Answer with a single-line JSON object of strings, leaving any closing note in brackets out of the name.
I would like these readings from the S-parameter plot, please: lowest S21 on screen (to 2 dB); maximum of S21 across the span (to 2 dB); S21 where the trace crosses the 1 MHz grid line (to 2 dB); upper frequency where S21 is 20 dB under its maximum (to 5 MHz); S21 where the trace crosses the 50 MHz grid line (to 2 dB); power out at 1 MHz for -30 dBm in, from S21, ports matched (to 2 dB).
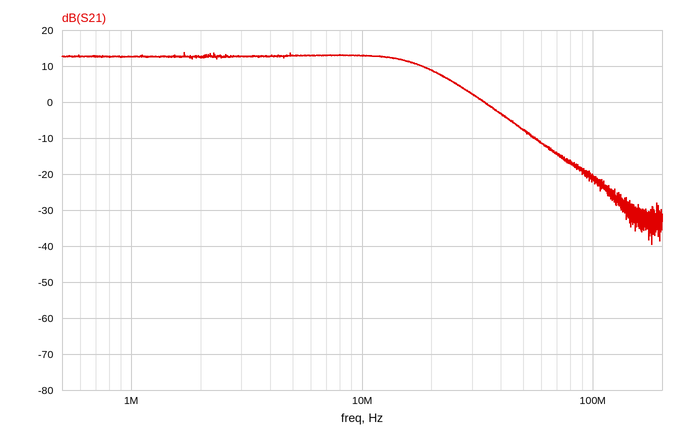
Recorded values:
{"lowest S21 on screen": "-40 dB", "maximum of S21 across the span": "14 dB", "S21 where the trace crosses the 1 MHz grid line": "12 dB", "upper frequency where S21 is 20 dB under its maximum": "45 MHz", "S21 where the trace crosses the 50 MHz grid line": "-8 dB", "power out at 1 MHz for -30 dBm in, from S21, ports matched": "-18 dBm"}
